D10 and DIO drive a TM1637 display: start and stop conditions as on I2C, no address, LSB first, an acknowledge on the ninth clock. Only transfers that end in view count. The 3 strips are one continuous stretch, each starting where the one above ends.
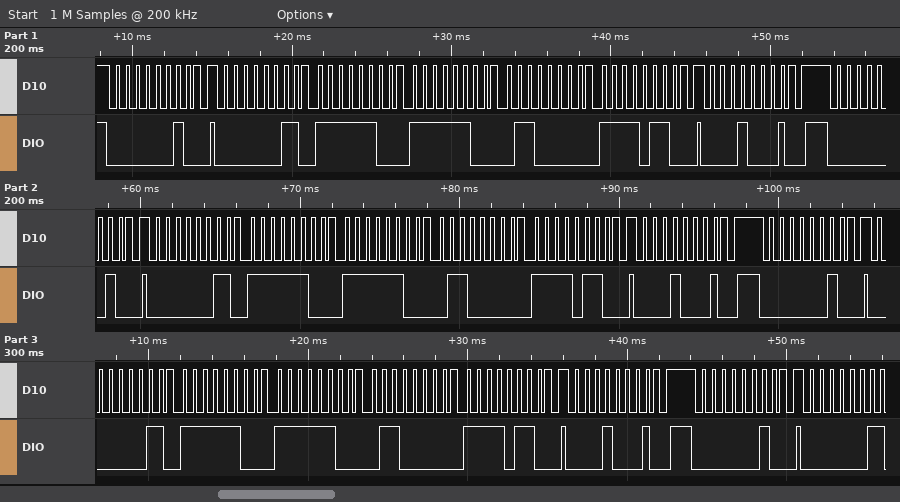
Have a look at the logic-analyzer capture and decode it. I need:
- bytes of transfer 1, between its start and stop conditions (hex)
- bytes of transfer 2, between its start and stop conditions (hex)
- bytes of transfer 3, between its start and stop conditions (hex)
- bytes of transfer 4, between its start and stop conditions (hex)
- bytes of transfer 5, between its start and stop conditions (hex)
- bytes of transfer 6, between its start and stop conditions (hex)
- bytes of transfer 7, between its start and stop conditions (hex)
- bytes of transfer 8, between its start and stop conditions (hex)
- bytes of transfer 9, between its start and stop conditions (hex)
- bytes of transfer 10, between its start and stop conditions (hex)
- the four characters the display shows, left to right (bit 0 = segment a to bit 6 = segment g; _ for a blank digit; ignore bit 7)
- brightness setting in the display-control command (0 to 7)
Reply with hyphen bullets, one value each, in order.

- 40
- C0 3F 3F 06 6F
- 88
- 40
- C0 3F 3F 06 6F
- 88
- 40
- C0 3F 3F 06 6F
- 88
- 40
- 0019
- 0
